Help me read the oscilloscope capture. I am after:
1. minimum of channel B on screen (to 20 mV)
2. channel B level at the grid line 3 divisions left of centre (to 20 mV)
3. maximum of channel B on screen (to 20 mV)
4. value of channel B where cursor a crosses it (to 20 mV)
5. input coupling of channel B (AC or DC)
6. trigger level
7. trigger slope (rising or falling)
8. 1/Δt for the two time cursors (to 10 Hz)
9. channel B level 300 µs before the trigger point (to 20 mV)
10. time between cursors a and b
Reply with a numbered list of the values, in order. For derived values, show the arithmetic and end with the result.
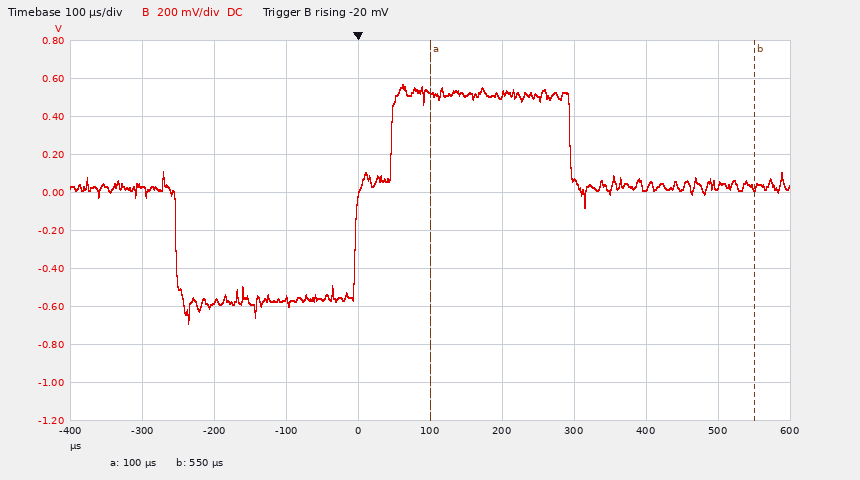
1. -680 mV
2. -580 mV
3. 560 mV
4. 520 mV
5. DC
6. -20 mV
7. rising
8. 1 / 450 µs ≈ 2.22 kHz
9. 40 mV
10. 550 µs − (100 µs) = 450 µs
